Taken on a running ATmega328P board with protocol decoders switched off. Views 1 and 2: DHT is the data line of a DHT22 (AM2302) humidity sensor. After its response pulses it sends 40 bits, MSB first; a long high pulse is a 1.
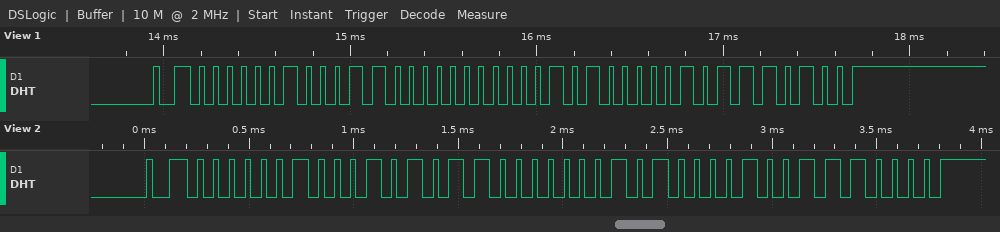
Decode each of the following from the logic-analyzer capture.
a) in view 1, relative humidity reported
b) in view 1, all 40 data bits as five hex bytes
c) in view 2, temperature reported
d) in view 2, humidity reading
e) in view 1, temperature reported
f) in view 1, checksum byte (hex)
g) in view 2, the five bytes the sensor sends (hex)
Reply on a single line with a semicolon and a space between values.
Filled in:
56.0 %; 02 30 01 41 74; 32.2 °C; 55.5 %; 32.1 °C; 0x74; 02 2B 01 42 70
